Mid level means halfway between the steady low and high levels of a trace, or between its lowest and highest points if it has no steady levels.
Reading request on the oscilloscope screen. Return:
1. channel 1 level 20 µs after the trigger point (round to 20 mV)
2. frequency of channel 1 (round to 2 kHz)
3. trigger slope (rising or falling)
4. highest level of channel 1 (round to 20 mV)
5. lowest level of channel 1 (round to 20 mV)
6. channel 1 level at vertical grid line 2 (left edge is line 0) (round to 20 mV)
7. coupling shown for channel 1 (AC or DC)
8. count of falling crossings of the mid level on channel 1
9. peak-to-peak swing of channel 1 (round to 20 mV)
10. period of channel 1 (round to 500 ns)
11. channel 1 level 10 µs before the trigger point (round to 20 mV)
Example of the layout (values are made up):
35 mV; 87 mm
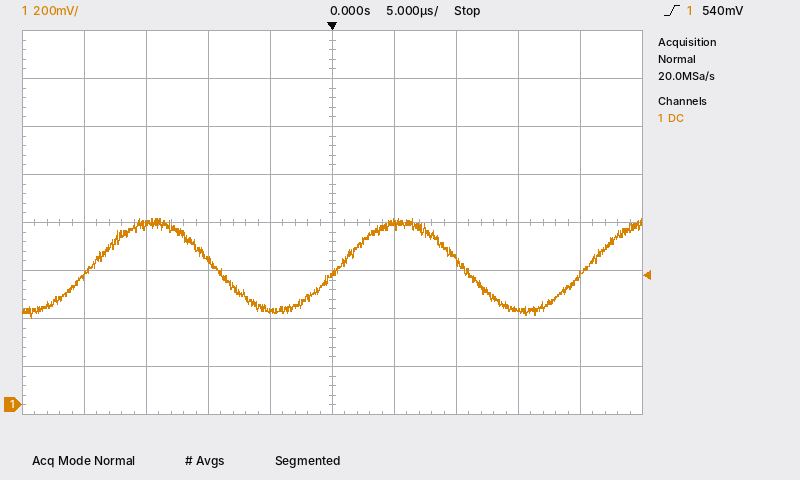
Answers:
540 mV; 50 kHz; rising; 780 mV; 360 mV; 740 mV; DC; 2; 420 mV; 20.0 µs; 600 mV
